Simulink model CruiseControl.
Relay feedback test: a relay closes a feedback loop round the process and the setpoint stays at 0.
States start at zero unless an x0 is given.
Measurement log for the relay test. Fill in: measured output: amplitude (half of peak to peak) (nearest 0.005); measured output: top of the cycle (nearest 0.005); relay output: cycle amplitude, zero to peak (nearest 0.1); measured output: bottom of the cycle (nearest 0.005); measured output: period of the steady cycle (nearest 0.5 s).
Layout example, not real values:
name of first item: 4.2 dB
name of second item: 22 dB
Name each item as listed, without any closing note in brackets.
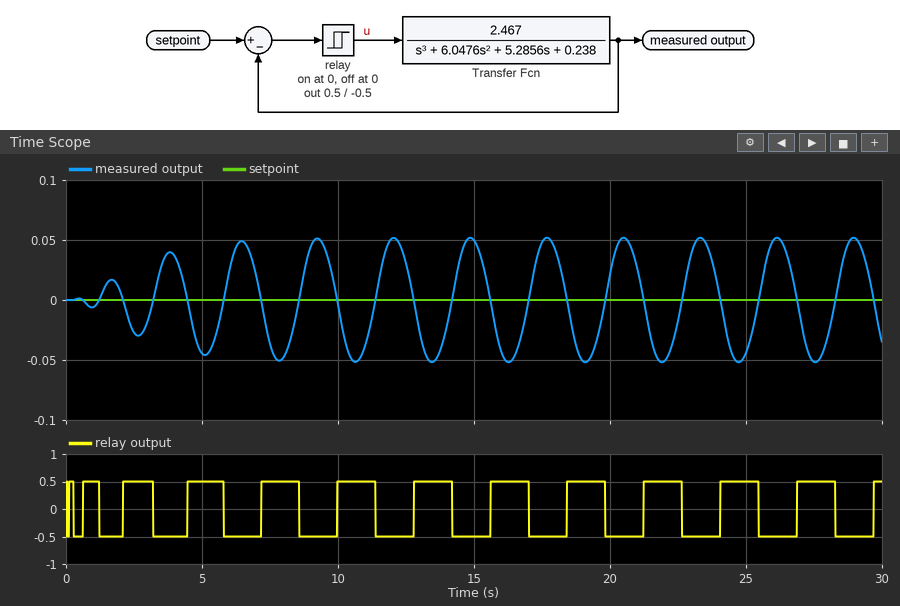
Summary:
measured output: amplitude (half of peak to peak): 0.050
measured output: top of the cycle: 0.050
relay output: cycle amplitude, zero to peak: 0.5
measured output: bottom of the cycle: -0.050
measured output: period of the steady cycle: 3.0 s
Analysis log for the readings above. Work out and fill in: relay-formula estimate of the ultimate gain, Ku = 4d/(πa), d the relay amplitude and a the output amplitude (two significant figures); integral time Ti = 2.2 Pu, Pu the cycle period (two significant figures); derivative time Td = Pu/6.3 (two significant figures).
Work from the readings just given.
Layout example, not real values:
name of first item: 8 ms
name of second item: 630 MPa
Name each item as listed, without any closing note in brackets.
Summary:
relay-formula estimate of the ultimate gain, Ku = 4d/(πa), d the relay amplitude and a the output amplitude: 13
integral time Ti = 2.2 Pu, Pu the cycle period: 6.6 s
derivative time Td = Pu/6.3: 0.48 s
